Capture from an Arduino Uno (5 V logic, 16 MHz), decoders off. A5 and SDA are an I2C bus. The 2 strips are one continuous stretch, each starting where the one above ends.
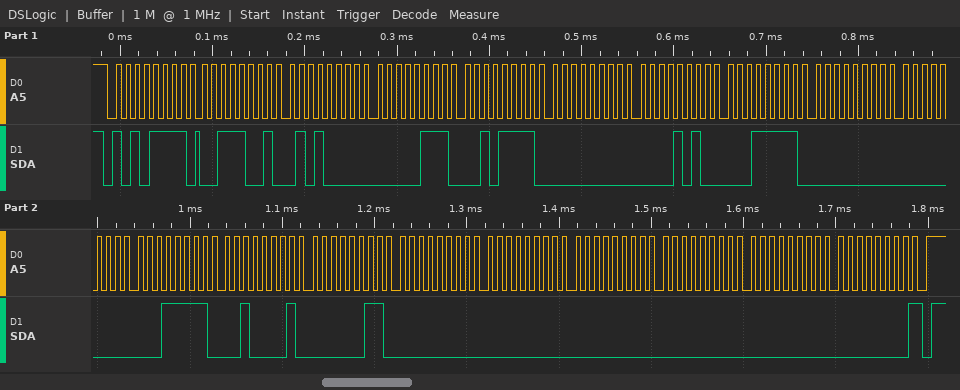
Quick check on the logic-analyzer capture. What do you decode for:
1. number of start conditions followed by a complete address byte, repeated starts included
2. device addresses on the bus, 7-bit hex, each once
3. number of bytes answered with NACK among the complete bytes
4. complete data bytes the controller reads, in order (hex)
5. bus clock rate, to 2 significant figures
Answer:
1
0x57
1
39 50 07 2F 00 0A 1F 00 00 1F 21 03 00 00 00 00 00 00
100 kHz
